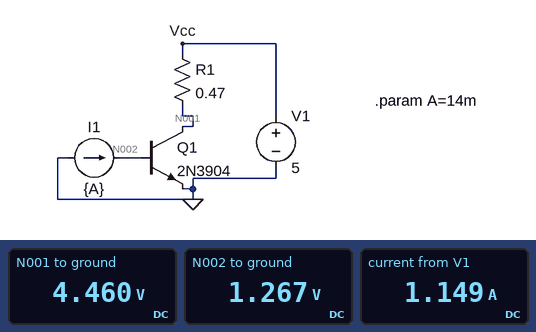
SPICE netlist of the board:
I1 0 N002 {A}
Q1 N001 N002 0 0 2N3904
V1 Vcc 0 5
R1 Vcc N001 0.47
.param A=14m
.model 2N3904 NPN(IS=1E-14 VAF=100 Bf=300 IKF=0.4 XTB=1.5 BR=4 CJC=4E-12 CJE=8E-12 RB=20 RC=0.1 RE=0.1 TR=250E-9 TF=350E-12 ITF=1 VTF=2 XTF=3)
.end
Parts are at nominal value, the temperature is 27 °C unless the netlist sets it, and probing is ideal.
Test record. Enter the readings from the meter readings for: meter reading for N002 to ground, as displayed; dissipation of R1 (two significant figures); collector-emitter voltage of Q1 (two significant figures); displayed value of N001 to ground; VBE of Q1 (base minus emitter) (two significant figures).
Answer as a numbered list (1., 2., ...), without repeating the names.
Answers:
1. 1.267 V
2. 620 mW
3. 4.5 V
4. 4.460 V
5. 1.3 V
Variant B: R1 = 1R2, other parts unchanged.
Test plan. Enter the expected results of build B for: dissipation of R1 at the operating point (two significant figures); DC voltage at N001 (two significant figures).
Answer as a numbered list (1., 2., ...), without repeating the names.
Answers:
1. 1.6 W
2. 3.6 V
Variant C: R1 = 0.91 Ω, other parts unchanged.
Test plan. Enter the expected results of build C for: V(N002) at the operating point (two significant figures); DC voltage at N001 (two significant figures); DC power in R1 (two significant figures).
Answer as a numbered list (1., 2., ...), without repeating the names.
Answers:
1. 1.3 V
2. 4.0 V
3. 1.2 W
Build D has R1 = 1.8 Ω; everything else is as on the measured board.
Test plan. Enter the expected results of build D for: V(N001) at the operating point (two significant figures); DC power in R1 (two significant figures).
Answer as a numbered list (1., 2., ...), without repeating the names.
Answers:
1. 3.0 V
2. 2.3 W
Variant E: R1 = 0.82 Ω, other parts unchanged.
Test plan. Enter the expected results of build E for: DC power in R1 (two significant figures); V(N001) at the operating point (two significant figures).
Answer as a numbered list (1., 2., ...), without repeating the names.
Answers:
1. 1.1 W
2. 4.1 V
